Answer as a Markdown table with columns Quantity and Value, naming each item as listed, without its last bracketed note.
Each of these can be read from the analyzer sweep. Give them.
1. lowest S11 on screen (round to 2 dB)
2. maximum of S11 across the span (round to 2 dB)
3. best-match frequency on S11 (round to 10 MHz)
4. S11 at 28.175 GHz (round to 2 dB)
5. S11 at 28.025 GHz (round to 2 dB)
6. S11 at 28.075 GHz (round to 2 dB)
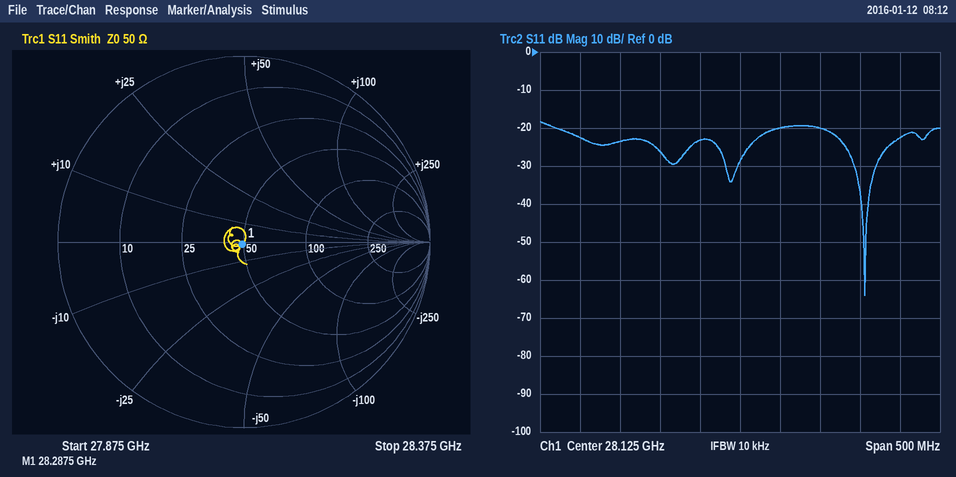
| Quantity | Value |
|---|---|
| lowest S11 on screen | -64 dB |
| maximum of S11 across the span | -18 dB |
| best-match frequency on S11 | 28.28 GHz |
| S11 at 28.175 GHz | -20 dB |
| S11 at 28.025 GHz | -26 dB |
| S11 at 28.075 GHz | -24 dB |
